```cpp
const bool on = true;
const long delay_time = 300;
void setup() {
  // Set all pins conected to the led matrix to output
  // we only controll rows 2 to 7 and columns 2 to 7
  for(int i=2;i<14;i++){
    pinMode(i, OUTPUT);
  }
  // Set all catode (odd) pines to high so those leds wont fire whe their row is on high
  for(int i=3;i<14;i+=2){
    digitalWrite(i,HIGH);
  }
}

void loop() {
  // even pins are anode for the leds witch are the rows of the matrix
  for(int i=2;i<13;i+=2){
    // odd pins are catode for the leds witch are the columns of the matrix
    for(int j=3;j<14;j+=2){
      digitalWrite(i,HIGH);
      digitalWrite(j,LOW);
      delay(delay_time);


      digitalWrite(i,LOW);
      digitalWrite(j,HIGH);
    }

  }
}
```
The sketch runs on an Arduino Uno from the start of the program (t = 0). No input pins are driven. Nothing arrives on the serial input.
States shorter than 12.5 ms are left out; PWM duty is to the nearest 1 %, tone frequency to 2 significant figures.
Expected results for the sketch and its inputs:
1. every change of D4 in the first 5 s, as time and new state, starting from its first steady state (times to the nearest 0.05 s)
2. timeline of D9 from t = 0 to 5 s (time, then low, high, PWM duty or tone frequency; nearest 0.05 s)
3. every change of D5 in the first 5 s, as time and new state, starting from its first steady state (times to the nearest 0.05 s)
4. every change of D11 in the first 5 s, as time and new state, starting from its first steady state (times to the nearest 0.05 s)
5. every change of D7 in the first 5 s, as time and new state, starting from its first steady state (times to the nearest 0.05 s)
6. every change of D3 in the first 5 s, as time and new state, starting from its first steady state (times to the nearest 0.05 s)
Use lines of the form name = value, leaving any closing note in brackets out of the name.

every change of D4 in the first 5 s, as time and new state, starting from its first steady state = 0 s low; 1.8 s high; 3.6 s low
timeline of D9 from t = 0 to 5 s = 0 s high; 0.9 s low; 1.2 s high; 2.7 s low; 3 s high; 4.5 s low; 4.8 s high
every change of D5 in the first 5 s, as time and new state, starting from its first steady state = 0 s high; 0.3 s low; 0.6 s high; 2.1 s low; 2.4 s high; 3.9 s low; 4.2 s high
every change of D11 in the first 5 s, as time and new state, starting from its first steady state = 0 s high; 1.2 s low; 1.5 s high; 3 s low; 3.3 s high; 4.8 s low
every change of D7 in the first 5 s, as time and new state, starting from its first steady state = 0 s high; 0.6 s low; 0.9 s high; 2.4 s low; 2.7 s high; 4.2 s low; 4.5 s high
every change of D3 in the first 5 s, as time and new state, starting from its first steady state = 0 s low; 0.3 s high; 1.8 s low; 2.1 s high; 3.6 s low; 3.9 s high
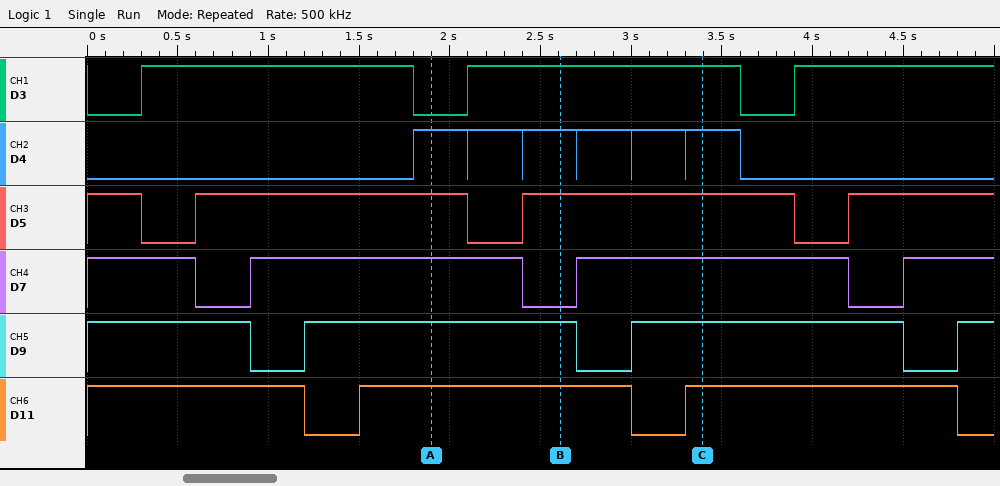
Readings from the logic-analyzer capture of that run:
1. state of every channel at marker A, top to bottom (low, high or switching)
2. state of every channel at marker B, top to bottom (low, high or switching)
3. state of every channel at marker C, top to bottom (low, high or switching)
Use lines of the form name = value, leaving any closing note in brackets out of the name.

state of every channel at marker A, top to bottom = D3 low, D4 high, D5 high, D7 high, D9 high, D11 high
state of every channel at marker B, top to bottom = D3 high, D4 high, D5 high, D7 low, D9 high, D11 high
state of every channel at marker C, top to bottom = D3 high, D4 high, D5 high, D7 high, D9 high, D11 high
